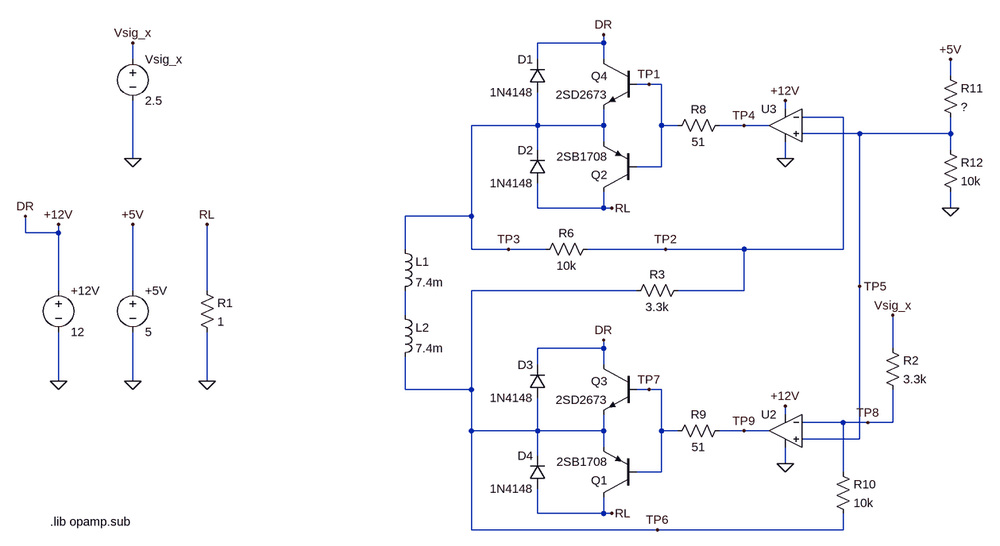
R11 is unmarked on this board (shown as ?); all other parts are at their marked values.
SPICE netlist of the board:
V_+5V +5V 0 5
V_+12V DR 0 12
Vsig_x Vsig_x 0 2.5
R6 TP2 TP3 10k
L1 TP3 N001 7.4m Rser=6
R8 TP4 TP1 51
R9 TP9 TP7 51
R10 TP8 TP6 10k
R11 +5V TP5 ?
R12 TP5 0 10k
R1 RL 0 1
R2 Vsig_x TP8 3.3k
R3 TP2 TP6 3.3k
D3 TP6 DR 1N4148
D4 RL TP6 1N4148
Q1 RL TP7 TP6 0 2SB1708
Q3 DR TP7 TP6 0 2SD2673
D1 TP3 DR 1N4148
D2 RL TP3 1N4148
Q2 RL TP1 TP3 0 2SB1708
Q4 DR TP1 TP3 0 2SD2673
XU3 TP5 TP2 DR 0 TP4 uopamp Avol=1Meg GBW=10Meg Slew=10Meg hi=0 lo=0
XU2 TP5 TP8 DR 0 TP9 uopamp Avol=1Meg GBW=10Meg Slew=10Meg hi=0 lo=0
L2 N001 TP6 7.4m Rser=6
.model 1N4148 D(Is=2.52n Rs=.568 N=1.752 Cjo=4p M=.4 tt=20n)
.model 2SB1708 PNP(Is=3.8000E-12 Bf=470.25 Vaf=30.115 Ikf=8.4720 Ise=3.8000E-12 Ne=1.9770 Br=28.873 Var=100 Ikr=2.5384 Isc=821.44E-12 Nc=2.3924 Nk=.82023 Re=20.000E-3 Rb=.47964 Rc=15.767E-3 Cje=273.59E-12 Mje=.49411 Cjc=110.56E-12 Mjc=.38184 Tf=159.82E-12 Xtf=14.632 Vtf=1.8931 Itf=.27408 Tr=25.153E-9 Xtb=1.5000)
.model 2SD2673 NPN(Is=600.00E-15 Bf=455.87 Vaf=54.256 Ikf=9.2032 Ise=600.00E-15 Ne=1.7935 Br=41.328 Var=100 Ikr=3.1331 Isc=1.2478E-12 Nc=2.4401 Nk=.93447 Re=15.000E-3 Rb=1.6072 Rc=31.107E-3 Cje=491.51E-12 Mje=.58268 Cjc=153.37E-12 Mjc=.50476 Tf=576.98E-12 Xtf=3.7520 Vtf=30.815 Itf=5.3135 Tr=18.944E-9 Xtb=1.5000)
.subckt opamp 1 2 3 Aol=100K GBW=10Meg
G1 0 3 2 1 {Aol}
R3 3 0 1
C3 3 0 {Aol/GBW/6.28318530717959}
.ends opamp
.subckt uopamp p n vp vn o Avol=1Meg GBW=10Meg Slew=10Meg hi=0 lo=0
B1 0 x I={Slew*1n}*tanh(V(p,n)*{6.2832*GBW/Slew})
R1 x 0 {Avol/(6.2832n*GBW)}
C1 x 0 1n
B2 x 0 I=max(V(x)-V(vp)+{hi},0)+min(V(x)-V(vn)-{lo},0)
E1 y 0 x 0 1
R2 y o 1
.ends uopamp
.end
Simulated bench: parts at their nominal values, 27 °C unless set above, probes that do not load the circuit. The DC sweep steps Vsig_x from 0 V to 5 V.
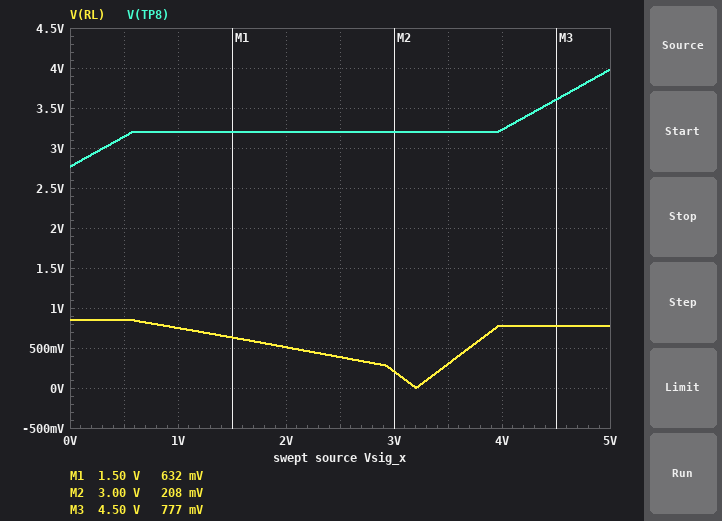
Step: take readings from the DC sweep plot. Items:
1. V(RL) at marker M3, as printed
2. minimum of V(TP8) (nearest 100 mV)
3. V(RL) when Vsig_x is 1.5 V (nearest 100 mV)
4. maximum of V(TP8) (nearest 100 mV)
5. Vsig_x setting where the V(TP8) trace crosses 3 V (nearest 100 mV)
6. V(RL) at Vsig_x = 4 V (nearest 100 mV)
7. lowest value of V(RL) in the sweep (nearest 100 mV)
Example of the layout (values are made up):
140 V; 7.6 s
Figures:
777 mV; 2.8 V; 600 mV; 4.0 V; 300 mV; 800 mV; 0 V
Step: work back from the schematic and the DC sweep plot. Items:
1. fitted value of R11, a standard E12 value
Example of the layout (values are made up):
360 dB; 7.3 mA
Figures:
5.6 kΩ
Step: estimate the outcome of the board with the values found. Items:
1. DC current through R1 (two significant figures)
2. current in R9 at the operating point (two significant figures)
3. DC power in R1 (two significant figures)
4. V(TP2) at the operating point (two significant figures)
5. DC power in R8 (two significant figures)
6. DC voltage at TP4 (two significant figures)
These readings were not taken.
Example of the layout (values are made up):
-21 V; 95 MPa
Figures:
390 mA; 830 µA; 150 mW; 4.2 V; 42 µW; -9.1 mV
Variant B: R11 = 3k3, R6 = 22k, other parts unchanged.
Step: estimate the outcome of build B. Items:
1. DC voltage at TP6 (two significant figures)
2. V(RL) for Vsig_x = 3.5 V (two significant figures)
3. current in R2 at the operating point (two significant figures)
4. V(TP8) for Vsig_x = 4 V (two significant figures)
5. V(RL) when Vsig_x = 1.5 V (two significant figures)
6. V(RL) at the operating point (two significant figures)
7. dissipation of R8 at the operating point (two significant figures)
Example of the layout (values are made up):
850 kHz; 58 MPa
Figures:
7.6 V; 320 mV; 380 µA; 3.8 V; 800 mV; 570 mV; 110 µW
